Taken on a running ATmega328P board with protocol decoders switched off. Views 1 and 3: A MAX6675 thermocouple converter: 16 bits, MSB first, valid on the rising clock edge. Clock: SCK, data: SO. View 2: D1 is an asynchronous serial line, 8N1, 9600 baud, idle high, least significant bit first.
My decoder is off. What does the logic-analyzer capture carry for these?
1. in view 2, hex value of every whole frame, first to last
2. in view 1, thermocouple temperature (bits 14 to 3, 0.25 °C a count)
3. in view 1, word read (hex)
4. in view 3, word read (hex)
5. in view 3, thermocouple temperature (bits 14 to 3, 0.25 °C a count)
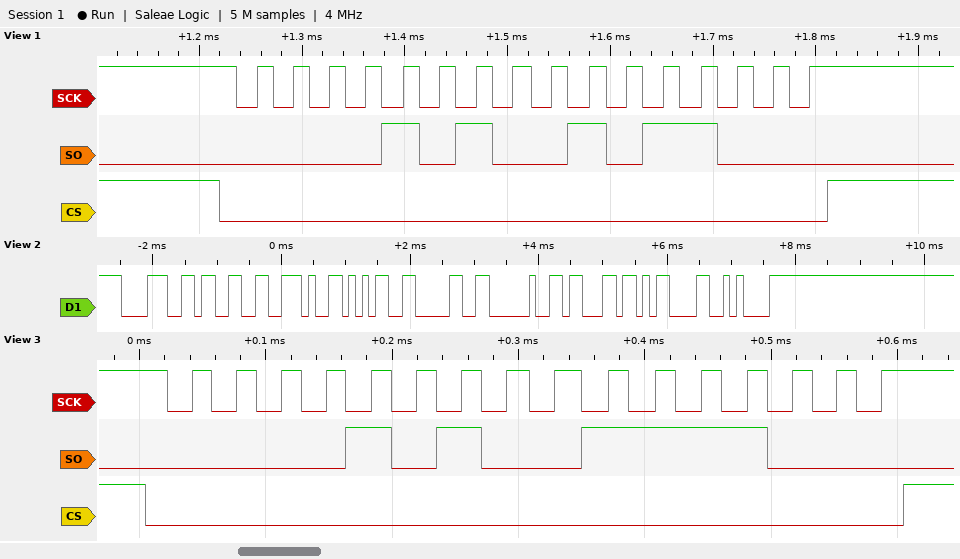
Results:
38 33 2E 35 30 20 63 0D 0A
82.75 °C
0x0A58
0x0A78
83.75 °C
